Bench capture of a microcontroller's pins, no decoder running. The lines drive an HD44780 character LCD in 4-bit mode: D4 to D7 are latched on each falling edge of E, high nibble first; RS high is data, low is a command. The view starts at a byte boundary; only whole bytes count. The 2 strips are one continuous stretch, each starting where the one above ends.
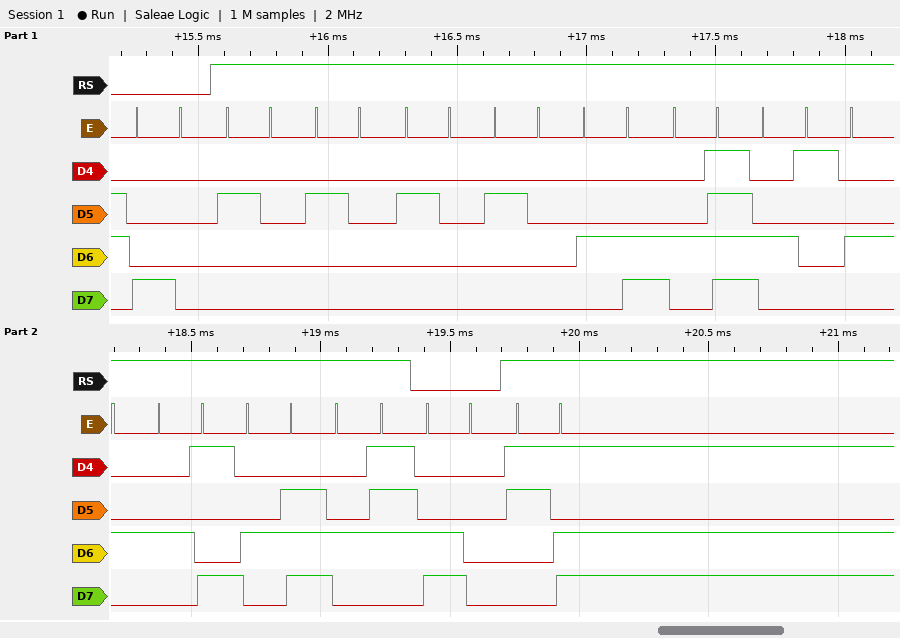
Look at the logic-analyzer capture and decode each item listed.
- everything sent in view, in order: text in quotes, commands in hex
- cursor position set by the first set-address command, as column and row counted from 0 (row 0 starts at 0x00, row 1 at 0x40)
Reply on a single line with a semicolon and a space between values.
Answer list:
0x80 "    LOADING" 0xC0 "="; column 0, row 0
